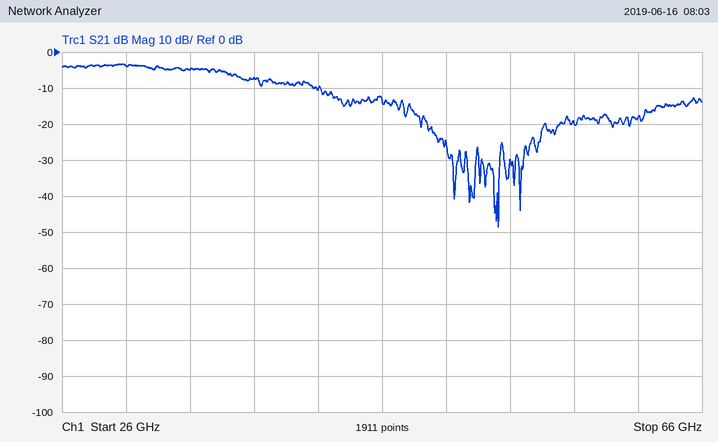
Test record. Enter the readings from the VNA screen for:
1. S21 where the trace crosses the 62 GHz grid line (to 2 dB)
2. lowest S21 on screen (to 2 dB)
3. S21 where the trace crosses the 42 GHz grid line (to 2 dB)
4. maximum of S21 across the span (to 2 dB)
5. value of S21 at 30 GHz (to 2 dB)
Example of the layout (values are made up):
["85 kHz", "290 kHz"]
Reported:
["-18 dB", "-48 dB", "-10 dB", "-4 dB", "-4 dB"]
